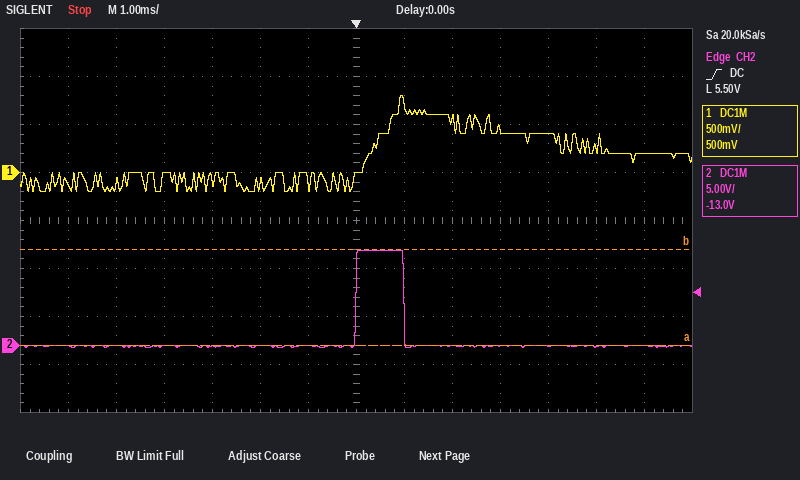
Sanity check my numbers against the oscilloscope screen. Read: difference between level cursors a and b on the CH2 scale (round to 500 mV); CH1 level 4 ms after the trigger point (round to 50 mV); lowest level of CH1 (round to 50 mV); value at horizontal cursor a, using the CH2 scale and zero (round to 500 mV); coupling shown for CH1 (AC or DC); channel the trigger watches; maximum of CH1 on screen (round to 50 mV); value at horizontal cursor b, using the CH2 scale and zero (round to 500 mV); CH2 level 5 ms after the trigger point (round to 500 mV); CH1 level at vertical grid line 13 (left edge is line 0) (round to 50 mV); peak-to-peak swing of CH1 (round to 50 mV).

10.0 V
400 mV
-200 mV
0.0 V
DC
CH2
800 mV
10.0 V
0.0 V
200 mV
1.00 V
